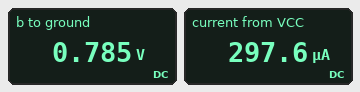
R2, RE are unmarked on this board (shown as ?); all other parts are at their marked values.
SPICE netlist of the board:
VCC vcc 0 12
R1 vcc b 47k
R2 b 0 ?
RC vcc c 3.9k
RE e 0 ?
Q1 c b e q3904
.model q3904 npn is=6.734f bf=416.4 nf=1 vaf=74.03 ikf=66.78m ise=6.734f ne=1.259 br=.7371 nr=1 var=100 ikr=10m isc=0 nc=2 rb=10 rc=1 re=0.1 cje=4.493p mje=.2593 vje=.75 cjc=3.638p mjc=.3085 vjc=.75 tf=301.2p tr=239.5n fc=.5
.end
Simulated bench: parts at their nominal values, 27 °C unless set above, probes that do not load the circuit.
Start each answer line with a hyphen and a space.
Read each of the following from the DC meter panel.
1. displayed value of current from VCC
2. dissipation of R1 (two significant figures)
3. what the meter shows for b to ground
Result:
- 297.6 µA
- 2.7 mW
- 0.785 V
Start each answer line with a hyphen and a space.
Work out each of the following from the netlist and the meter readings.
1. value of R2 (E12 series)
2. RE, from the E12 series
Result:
- 3.3 kΩ
- 3.3 kΩ
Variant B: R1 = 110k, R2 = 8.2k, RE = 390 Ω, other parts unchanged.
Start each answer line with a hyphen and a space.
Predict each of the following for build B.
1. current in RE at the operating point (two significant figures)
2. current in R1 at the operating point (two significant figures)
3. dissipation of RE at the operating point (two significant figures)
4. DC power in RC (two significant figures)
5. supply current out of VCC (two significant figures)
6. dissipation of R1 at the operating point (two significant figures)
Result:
- 430 µA
- 100 µA
- 72 µW
- 710 µW
- 530 µA
- 1.1 mW
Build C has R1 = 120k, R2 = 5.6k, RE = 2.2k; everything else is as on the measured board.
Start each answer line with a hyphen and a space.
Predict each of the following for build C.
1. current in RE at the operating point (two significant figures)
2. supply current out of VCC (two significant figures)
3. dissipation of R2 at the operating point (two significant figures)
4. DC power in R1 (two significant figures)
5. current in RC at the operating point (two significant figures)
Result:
- 4.9 µA
- 100 µA
- 51 µW
- 1.1 mW
- 4.8 µA
